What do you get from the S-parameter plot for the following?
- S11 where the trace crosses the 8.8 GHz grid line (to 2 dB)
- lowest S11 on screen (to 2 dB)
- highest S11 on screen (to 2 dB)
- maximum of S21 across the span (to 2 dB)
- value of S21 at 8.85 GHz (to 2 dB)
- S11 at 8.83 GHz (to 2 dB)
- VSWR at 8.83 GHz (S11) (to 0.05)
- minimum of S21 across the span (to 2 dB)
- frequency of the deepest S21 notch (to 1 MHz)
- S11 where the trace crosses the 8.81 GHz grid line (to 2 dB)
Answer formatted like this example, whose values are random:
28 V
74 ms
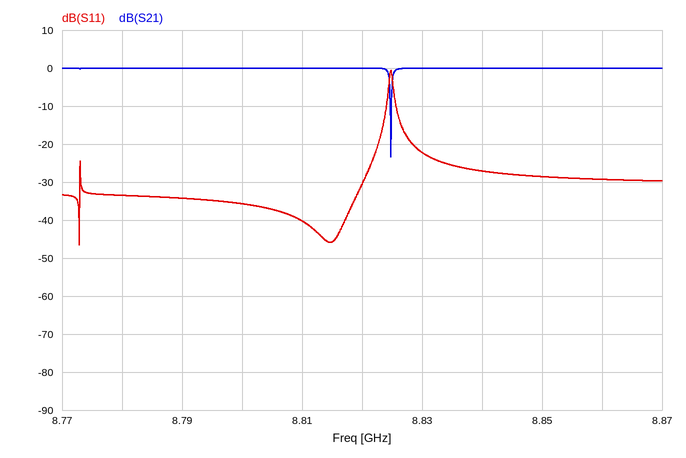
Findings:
-36 dB
-46 dB
0 dB
0 dB
0 dB
-22 dB
1.15
-24 dB
8.825 GHz
-40 dB
